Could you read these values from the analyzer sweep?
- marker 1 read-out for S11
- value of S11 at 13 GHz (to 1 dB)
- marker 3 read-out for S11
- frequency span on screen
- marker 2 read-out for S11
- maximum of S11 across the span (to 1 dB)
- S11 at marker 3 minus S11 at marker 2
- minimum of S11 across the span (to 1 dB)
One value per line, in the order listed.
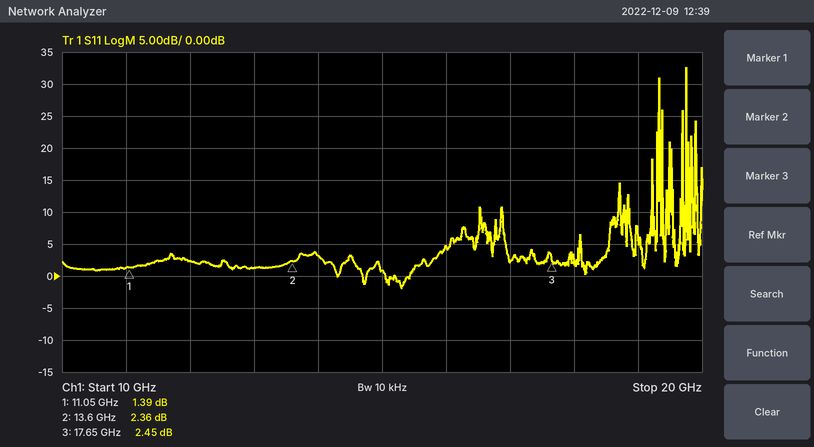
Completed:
1.39 dB
1 dB
2.45 dB
10 GHz
2.36 dB
33 dB
0.09 dB
-2 dB
